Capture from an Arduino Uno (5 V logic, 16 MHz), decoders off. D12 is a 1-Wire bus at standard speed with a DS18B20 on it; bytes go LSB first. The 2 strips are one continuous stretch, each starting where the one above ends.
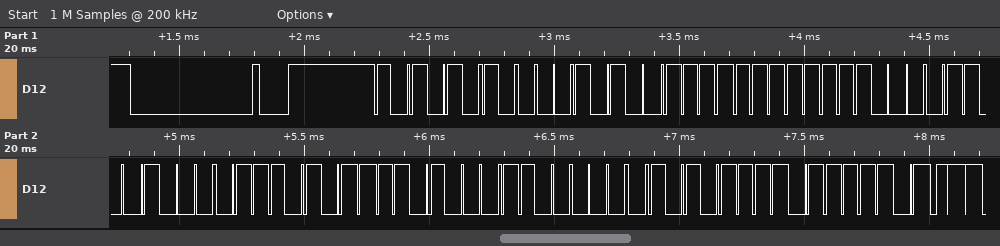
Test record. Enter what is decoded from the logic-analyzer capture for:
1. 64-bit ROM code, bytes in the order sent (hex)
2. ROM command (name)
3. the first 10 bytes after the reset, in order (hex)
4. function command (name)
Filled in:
28 FF 0F 13 AE 17 03 F5
Match ROM
55 28 FF 0F 13 AE 17 03 F5 BE
Read Scratchpad
